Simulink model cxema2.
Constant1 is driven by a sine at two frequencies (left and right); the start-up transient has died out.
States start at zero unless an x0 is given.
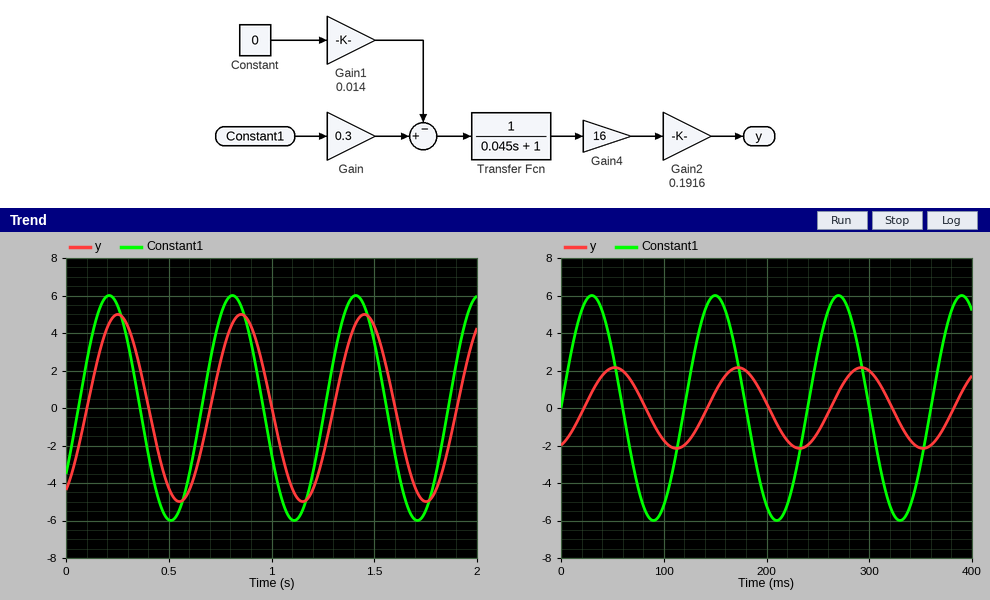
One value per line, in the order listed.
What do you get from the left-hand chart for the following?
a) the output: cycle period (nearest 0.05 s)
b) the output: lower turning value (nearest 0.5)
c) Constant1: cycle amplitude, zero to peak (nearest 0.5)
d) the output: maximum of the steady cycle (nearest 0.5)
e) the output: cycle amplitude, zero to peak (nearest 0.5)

0.60 s
-5.0
6.0
5.0
5.0
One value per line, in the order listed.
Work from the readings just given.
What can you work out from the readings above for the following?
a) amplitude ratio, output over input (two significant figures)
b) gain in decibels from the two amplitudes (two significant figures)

0.83
-1.6 dB
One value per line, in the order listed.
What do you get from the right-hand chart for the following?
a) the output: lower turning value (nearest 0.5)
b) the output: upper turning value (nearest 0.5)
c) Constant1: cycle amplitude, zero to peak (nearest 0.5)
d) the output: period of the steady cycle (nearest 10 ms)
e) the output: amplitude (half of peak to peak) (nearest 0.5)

-2.0
2.0
6.0
120 ms
2.0
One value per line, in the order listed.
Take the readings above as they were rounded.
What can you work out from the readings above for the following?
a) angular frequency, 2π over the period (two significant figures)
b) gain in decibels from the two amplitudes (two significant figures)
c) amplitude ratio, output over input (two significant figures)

0.052 rad/ms
-9.5 dB
0.33
